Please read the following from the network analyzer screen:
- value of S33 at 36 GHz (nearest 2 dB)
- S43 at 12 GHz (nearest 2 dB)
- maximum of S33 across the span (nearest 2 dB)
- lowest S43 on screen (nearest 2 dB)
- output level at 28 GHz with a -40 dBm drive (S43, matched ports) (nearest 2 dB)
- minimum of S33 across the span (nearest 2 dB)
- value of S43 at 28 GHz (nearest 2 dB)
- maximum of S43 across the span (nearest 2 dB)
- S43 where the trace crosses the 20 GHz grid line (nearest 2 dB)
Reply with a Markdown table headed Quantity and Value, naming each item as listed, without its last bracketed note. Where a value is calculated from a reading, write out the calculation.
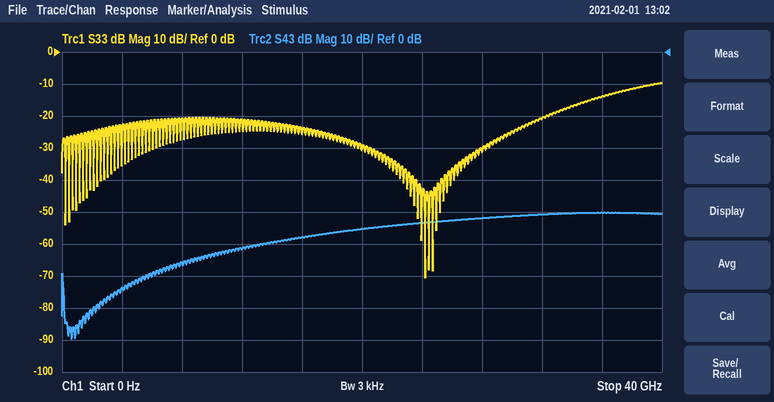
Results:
| Quantity | Value |
|---|---|
| value of S33 at 36 GHz | -14 dB |
| S43 at 12 GHz | -62 dB |
| maximum of S33 across the span | -10 dB |
| lowest S43 on screen | -90 dB |
| output level at 28 GHz with a -40 dBm drive (S43, matched ports) | -40 dBm + (-52 dB) = -92 dBm |
| minimum of S33 across the span | -70 dB |
| value of S43 at 28 GHz | -52 dB |
| maximum of S43 across the span | -50 dB |
| S43 where the trace crosses the 20 GHz grid line | -56 dB |
